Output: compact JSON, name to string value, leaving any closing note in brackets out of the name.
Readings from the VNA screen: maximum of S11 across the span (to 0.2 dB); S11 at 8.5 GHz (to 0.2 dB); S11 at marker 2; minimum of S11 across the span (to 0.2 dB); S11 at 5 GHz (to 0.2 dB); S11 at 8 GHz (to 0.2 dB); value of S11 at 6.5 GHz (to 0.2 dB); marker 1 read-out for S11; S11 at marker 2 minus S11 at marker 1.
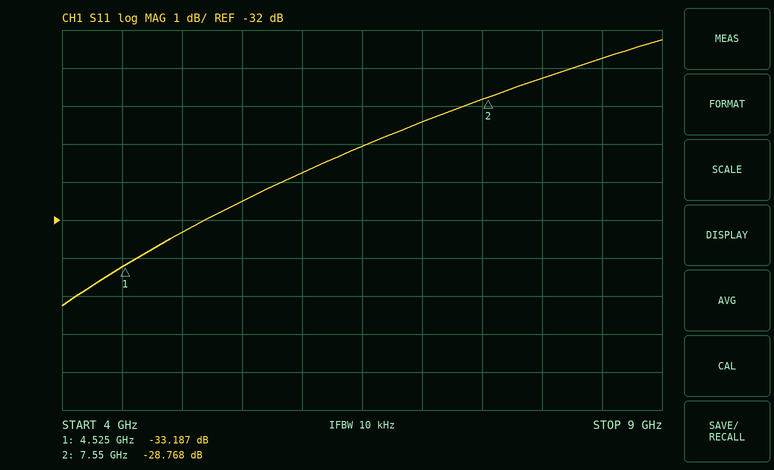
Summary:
{"maximum of S11 across the span": "-27.2 dB", "S11 at 8.5 GHz": "-27.8 dB", "S11 at marker 2": "-28.768 dB", "minimum of S11 across the span": "-34.2 dB", "S11 at 5 GHz": "-32.4 dB", "S11 at 8 GHz": "-28.2 dB", "value of S11 at 6.5 GHz": "-30.0 dB", "marker 1 read-out for S11": "-33.187 dB", "S11 at marker 2 minus S11 at marker 1": "4.419 dB"}
